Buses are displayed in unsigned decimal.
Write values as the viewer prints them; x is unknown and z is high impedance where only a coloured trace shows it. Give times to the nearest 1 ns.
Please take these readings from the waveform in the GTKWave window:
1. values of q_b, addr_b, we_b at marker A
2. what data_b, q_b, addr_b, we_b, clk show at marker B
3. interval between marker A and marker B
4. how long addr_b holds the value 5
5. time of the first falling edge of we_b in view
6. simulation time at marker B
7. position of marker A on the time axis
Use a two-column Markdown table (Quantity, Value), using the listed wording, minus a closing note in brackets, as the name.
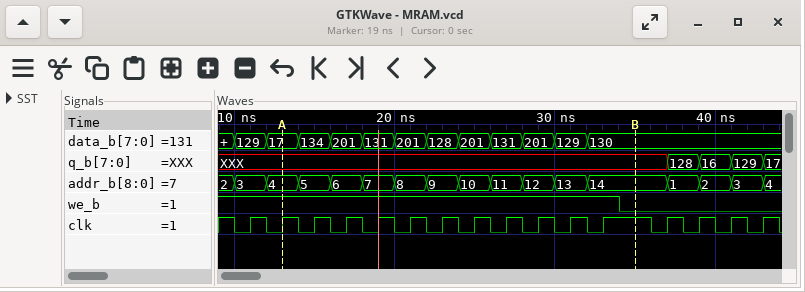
| Quantity | Value |
|---|---|
| values of q_b, addr_b, we_b at marker A | q_b=XXX, addr_b=4, we_b=1 |
| what data_b, q_b, addr_b, we_b, clk show at marker B | data_b=130, q_b=XXX, addr_b=14, we_b=0, clk=1 |
| interval between marker A and marker B | 22 ns |
| how long addr_b holds the value 5 | 2 ns |
| time of the first falling edge of we_b in view | 34 ns |
| simulation time at marker B | 35 ns |
| position of marker A on the time axis | 13 ns |
